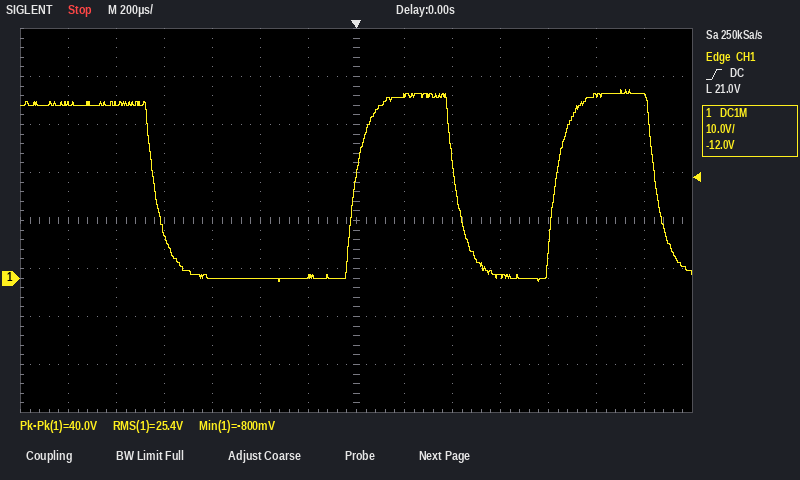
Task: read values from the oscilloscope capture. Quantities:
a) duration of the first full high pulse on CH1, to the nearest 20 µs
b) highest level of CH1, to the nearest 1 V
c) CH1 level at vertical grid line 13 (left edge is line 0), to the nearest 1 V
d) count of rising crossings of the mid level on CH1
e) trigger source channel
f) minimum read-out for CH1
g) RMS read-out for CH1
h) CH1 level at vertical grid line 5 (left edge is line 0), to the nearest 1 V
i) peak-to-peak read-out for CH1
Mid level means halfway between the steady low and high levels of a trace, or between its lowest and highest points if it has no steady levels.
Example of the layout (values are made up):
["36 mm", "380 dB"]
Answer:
["420 µs", "39 V", "38 V", "2", "CH1", "-800 mV", "25.4 V", "0 V", "40.0 V"]
